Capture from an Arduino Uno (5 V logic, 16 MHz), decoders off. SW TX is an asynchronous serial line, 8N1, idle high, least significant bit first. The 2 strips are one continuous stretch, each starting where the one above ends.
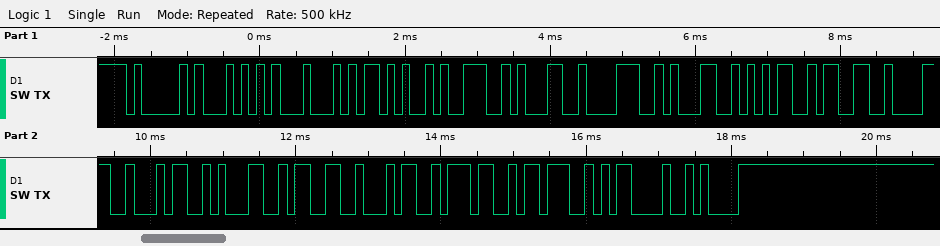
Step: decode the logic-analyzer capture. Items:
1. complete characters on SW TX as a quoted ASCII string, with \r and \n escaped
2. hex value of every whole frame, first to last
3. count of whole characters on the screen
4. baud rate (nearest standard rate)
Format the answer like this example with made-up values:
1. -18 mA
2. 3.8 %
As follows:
1. "ATD+918153841347;\r\n"
2. 0x41 0x54 0x44 0x2B 0x39 0x31 0x38 0x31 0x35 0x33 0x38 0x34 0x31 0x33 0x34 0x37 0x3B 0x0D 0x0A
3. 19
4. 9600 baud
